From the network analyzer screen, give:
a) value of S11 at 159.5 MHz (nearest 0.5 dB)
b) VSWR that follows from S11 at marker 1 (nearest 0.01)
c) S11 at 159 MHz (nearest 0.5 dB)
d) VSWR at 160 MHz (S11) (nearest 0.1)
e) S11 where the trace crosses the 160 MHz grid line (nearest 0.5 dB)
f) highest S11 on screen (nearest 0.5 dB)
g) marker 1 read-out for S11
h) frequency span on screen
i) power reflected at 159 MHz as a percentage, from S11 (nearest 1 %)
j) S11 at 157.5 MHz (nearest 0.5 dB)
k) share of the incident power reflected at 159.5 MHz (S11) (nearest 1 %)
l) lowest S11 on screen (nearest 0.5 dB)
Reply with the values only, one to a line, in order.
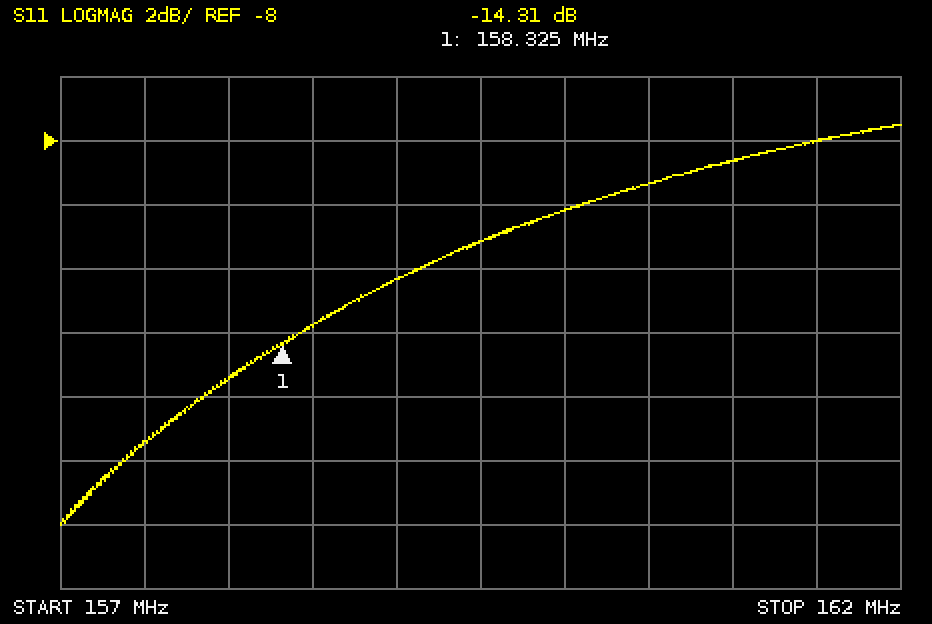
-11.0 dB
1.48
-12.5 dB
1.9
-10.0 dB
-7.5 dB
-14.31 dB
5 MHz
6 %
-17.5 dB
8 %
-20.0 dB
